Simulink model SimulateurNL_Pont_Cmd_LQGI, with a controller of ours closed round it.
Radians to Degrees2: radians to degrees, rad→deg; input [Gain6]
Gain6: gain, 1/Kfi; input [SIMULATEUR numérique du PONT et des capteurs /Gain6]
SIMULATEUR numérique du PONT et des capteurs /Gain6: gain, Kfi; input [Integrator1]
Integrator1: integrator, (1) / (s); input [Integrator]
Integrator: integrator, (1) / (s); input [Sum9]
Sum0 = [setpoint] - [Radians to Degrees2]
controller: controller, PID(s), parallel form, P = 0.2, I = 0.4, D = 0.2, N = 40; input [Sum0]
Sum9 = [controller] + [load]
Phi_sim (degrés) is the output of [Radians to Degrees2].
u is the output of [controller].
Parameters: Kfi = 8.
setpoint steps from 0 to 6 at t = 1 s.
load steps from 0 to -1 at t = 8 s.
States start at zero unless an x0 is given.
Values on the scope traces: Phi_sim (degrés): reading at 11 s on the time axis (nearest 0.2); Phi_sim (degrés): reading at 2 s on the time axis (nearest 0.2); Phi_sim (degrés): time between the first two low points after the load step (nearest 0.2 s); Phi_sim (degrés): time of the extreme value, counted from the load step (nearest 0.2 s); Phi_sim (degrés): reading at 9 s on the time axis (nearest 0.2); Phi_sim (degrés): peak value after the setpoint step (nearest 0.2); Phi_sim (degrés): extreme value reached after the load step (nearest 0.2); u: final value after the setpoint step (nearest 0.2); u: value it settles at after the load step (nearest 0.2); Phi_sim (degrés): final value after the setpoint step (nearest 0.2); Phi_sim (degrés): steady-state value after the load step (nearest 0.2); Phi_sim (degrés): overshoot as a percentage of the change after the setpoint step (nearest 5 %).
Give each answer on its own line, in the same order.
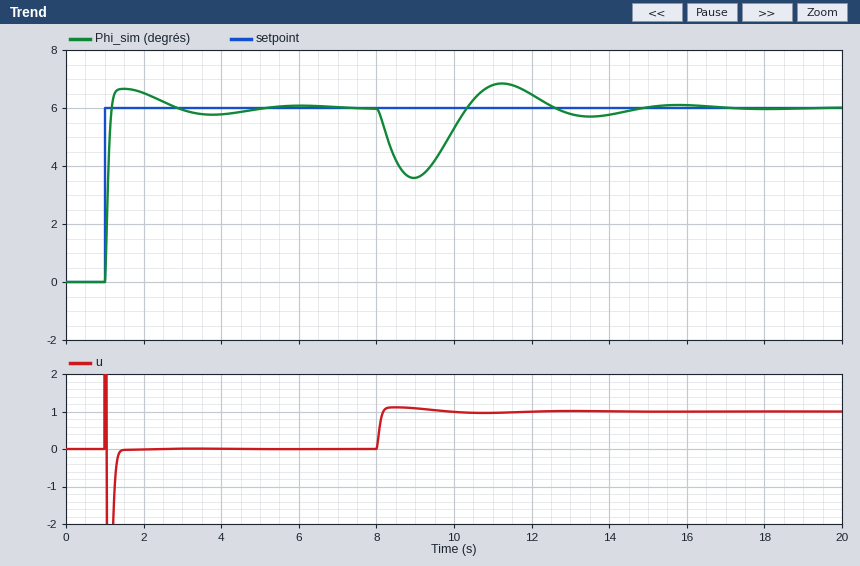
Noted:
6.8
6.6
4.6 s
1.0 s
3.6
6.6
3.6
0.0
1.0
6.0
6.0
10 %
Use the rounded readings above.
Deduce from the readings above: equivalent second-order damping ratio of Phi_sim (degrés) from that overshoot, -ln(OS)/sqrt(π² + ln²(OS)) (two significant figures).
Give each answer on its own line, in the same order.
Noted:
0.59
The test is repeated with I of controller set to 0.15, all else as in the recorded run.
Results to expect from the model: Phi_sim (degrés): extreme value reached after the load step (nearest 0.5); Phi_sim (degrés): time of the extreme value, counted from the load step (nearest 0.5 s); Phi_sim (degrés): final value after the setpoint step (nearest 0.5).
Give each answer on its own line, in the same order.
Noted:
3.0
1.5 s
6.0
